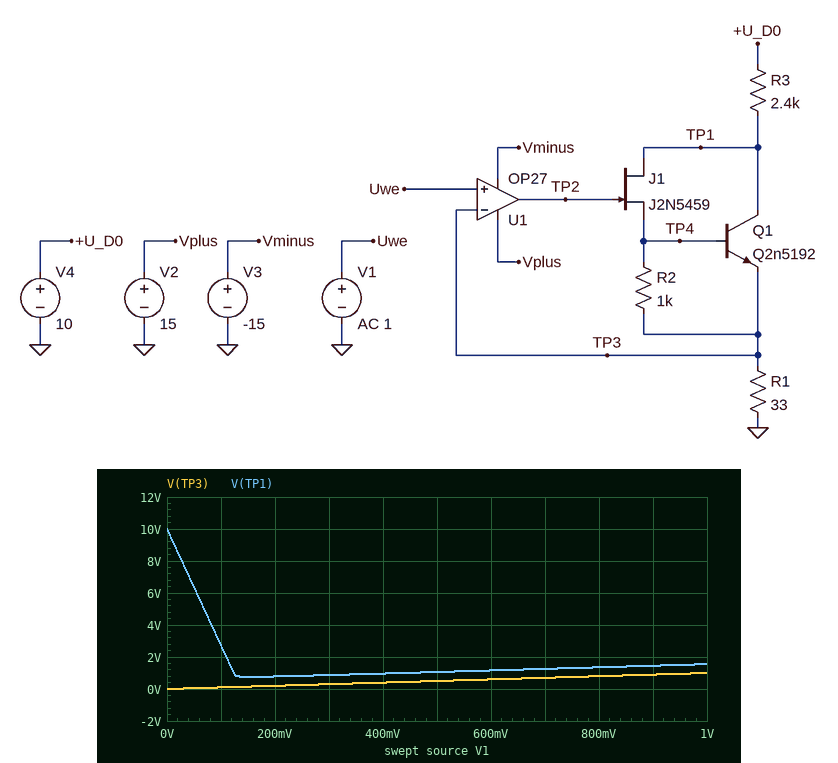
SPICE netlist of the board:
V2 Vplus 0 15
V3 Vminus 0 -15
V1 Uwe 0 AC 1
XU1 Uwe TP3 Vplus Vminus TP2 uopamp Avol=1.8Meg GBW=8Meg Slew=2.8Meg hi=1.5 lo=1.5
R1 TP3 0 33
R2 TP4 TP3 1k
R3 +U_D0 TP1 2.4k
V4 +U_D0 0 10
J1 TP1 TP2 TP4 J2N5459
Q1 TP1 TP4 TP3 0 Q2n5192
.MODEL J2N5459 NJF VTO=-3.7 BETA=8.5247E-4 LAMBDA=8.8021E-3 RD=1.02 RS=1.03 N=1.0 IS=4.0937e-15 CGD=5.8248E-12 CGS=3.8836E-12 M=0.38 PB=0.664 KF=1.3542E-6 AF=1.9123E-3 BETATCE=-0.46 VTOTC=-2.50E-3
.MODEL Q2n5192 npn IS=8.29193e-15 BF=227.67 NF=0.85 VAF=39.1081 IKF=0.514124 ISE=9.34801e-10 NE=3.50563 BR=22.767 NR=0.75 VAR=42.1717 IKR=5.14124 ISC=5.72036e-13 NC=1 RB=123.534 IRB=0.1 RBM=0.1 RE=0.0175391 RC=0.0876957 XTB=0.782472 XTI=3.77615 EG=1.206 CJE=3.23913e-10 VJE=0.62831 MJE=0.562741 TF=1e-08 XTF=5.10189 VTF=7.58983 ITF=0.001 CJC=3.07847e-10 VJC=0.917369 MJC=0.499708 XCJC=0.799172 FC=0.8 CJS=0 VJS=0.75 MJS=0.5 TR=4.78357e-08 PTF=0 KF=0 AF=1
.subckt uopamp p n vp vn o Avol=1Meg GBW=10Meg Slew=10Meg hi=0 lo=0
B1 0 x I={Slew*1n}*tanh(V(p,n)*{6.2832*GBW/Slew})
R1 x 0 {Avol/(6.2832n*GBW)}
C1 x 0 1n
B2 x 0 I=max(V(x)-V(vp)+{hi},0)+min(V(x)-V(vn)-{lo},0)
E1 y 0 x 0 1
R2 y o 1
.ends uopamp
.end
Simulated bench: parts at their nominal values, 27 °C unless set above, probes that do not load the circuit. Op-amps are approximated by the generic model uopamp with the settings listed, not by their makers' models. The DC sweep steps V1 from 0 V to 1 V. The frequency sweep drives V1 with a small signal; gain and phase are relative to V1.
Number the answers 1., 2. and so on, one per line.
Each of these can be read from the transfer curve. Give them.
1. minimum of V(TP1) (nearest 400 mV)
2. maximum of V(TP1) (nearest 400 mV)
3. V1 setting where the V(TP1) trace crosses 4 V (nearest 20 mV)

1. 800 mV
2. 10.0 V
3. 80 mV
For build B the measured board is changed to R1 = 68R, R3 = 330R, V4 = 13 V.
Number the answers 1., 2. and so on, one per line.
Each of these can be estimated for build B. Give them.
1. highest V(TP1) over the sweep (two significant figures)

1. 13 V
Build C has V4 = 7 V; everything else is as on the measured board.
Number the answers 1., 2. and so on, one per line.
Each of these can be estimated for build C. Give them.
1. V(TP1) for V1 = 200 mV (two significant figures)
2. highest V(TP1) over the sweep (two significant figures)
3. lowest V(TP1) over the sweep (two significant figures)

1. 770 mV
2. 7.0 V
3. 710 mV
